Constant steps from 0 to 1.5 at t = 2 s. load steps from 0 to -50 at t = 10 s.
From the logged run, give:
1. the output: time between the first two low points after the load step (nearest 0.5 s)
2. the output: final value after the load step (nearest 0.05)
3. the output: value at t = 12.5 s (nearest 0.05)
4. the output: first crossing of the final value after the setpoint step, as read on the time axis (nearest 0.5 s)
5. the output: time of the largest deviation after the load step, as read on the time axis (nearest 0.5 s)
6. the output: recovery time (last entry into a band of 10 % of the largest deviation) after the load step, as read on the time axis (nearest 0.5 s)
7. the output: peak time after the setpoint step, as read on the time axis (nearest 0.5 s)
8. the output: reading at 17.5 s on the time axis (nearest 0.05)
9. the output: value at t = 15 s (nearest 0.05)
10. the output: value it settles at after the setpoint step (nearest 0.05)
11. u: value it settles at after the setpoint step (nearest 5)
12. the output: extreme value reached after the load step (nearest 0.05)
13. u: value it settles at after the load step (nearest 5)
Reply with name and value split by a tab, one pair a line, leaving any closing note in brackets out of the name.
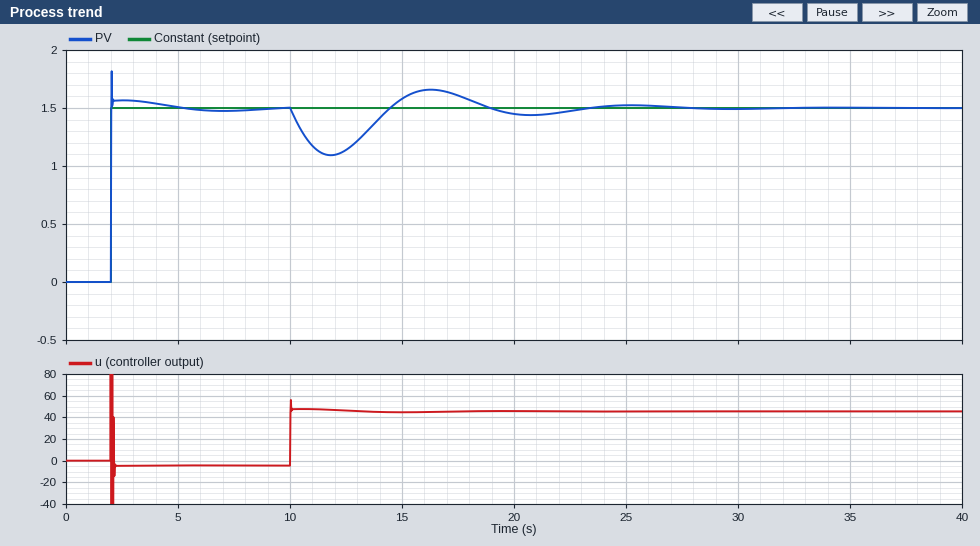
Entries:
the output: time between the first two low points after the load step	9.0 s
the output: final value after the load step	1.50
the output: value at t = 12.5 s	1.15
the output: first crossing of the final value after the setpoint step, as read on the time axis	2.0 s
the output: time of the largest deviation after the load step, as read on the time axis	12.0 s
the output: recovery time (last entry into a band of 10 % of the largest deviation) after the load step, as read on the time axis	22.0 s
the output: peak time after the setpoint step, as read on the time axis	2.0 s
the output: reading at 17.5 s on the time axis	1.60
the output: value at t = 15 s	1.60
the output: value it settles at after the setpoint step	1.50
u: value it settles at after the setpoint step	-5
the output: extreme value reached after the load step	1.10
u: value it settles at after the load step	45
